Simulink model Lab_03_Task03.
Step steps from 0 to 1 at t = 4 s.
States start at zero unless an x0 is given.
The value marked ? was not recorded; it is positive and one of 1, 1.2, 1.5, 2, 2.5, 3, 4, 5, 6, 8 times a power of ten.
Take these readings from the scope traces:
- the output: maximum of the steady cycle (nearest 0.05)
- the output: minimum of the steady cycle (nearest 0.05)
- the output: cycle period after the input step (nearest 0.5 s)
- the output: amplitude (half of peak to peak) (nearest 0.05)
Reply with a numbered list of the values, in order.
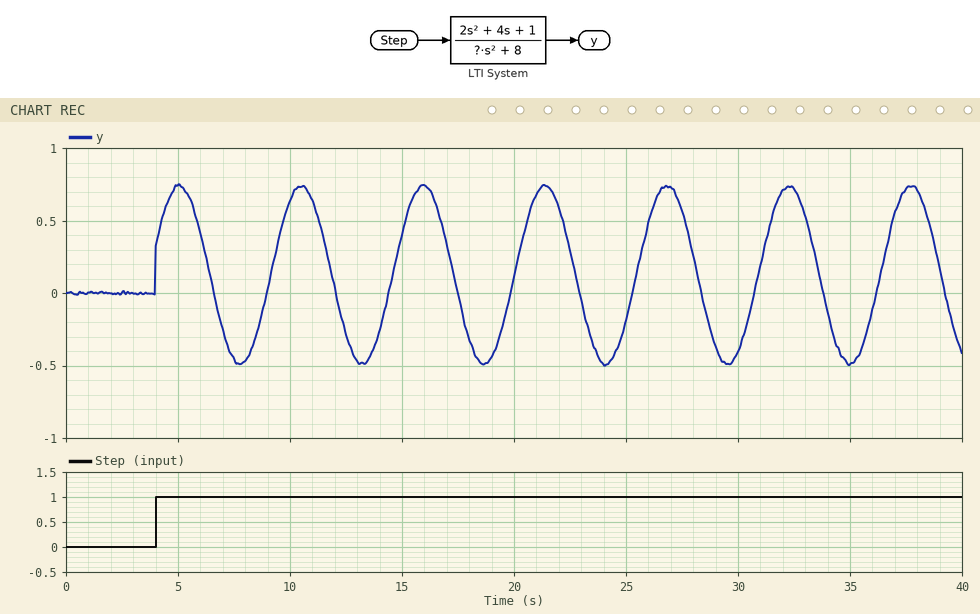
1. 0.75
2. -0.50
3. 5.5 s
4. 0.60
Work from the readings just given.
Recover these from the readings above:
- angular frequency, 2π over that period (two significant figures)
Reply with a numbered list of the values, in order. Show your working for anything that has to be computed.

1. 2π / 5.5 = 1.1 rad/s
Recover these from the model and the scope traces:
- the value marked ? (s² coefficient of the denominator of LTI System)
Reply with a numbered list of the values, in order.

1. 6
